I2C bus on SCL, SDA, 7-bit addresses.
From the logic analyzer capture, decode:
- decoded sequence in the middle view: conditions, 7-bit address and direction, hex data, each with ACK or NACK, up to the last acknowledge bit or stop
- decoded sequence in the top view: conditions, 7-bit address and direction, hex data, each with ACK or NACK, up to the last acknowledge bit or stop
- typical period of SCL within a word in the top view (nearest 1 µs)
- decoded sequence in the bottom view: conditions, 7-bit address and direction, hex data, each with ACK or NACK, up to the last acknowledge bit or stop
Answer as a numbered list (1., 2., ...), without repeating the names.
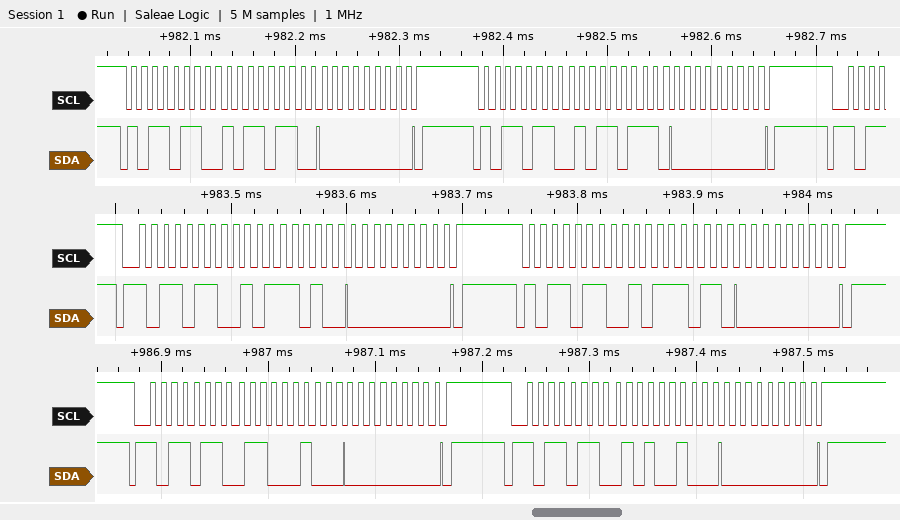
1. start, address 5B write ACK, BA ACK, 00 ACK, stop, start, address 5B write ACK, BB ACK, 00 ACK, stop
2. start, address 5B write ACK, B6 ACK, 00 ACK, stop, start, address 5B write ACK, B7 ACK, 00 ACK, stop
3. 10 µs
4. start, address 5B write ACK, C4 ACK, 00 ACK, stop, start, address 5B write ACK, A4 ACK, 00 ACK, stop
